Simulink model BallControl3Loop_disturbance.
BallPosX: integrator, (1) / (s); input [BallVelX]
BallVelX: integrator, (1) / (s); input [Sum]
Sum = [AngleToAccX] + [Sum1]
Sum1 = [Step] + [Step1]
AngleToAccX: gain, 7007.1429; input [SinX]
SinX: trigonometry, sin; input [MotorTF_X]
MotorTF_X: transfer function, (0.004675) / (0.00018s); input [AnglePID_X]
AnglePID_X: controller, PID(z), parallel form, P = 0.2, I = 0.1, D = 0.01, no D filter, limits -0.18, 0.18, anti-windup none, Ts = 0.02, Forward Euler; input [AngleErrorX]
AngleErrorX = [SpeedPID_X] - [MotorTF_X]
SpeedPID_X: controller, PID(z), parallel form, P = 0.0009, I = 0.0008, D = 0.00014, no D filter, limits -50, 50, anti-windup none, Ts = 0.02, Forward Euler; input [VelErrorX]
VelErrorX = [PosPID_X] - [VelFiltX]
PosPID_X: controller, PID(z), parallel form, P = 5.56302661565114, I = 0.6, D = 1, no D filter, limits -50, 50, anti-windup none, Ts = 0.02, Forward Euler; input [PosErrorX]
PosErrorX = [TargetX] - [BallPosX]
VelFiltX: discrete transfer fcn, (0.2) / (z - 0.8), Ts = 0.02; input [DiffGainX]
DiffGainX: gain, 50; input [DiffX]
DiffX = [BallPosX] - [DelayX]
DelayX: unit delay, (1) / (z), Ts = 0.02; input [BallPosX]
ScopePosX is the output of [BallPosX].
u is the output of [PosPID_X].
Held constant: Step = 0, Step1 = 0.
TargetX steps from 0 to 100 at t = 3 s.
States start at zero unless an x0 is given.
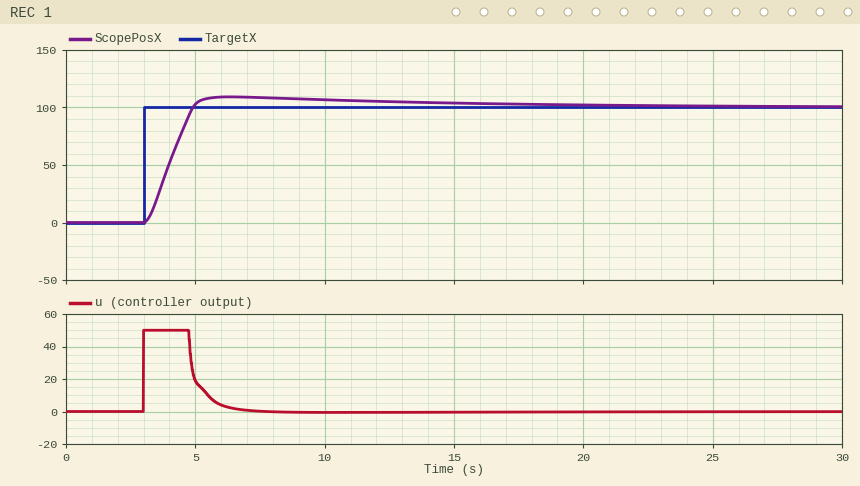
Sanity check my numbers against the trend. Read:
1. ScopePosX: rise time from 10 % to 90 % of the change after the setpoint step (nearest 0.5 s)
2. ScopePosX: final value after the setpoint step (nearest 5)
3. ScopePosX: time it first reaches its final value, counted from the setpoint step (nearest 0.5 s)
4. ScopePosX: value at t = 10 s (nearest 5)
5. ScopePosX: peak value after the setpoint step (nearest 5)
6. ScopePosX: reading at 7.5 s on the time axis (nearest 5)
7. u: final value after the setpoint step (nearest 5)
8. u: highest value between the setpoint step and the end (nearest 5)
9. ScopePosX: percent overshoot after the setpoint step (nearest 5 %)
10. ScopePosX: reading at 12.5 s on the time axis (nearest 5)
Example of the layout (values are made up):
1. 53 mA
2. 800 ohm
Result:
1. 1.5 s
2. 100
3. 2.0 s
4. 105
5. 110
6. 110
7. 0
8. 50
9. 10 %
10. 105
